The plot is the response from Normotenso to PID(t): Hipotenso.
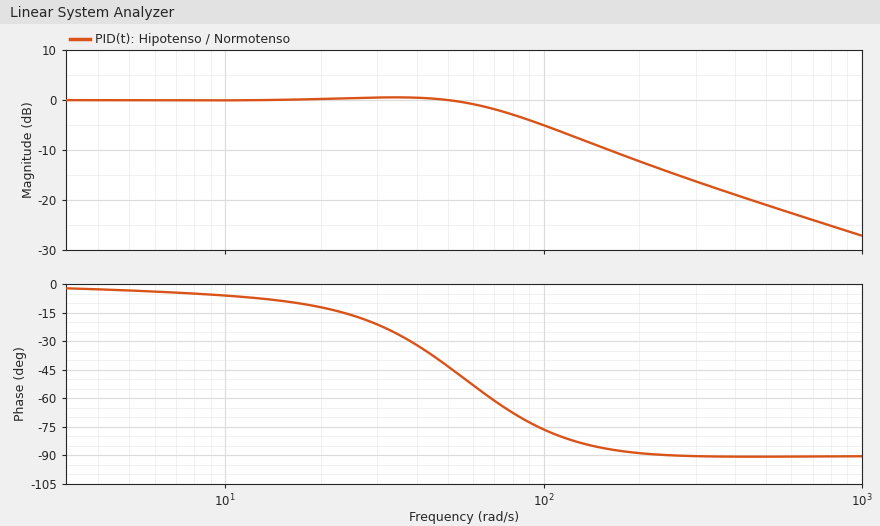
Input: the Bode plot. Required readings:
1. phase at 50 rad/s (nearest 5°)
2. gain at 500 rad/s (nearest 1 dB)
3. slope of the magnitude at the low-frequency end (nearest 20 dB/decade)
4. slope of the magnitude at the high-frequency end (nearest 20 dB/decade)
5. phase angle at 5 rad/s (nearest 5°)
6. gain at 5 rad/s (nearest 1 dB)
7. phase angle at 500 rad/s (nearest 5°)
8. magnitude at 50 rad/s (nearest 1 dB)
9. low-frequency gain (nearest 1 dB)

-45°
-21 dB
0 dB/decade
-20 dB/decade
-5°
0 dB
-90°
0 dB
0 dB
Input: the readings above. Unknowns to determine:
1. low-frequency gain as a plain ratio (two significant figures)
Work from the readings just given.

1.0
